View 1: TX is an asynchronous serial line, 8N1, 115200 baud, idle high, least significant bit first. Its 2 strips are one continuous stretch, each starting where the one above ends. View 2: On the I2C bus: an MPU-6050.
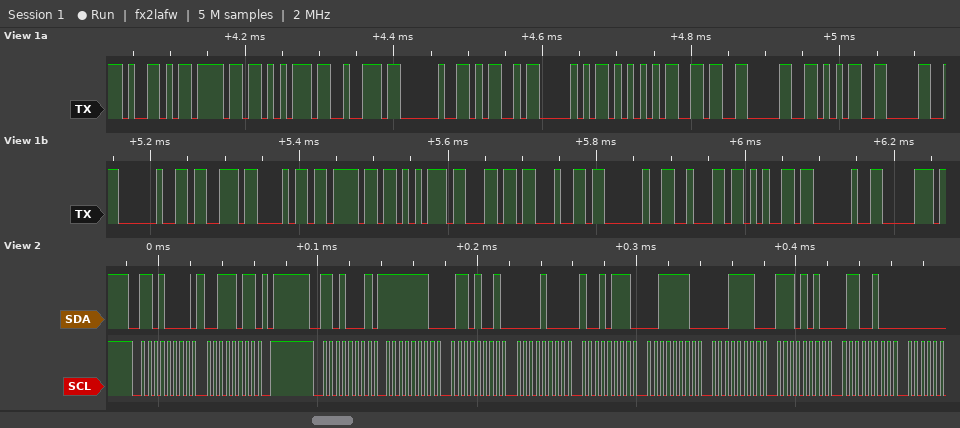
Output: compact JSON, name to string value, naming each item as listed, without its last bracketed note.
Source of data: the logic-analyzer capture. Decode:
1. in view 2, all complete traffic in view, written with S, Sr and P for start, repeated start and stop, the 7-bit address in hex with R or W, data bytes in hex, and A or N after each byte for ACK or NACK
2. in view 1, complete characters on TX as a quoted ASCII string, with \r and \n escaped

{"in view 2, all complete traffic in view, written with S, Sr and P for start, repeated start and stop, the 7-bit address in hex with R or W, data bytes in hex, and A or N after each byte for ACK or NACK": "S 68W A 3B A P S 68R A FE A 69 A 08 A 97 A 3E A 1E A EA A 64 A", "in view 1, complete characters on TX as a quoted ASCII string, with \\r and \\n escaped": "\"Your MPU6050 should be p\""}
